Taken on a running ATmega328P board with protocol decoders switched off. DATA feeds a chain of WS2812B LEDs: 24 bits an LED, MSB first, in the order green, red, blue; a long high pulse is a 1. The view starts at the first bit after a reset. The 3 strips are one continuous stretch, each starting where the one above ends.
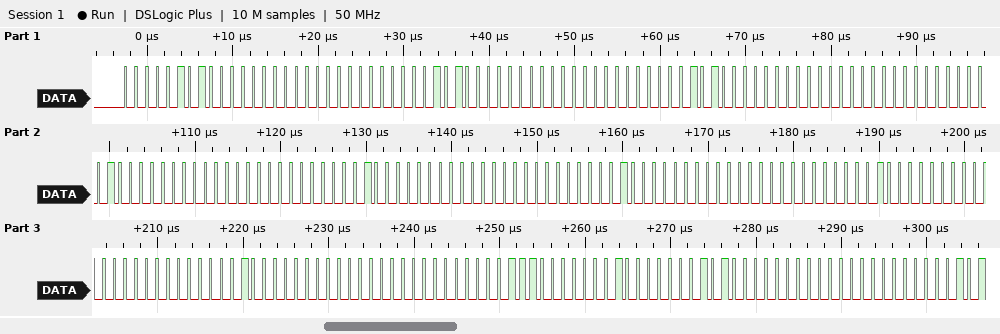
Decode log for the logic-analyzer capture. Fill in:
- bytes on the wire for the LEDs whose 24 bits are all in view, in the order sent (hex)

05 00 00 05 00 00 05 00 00 00 20 00 00 20 00 00 20 00 00 20 00 00 20 00 00 1C 04 05 00 00
